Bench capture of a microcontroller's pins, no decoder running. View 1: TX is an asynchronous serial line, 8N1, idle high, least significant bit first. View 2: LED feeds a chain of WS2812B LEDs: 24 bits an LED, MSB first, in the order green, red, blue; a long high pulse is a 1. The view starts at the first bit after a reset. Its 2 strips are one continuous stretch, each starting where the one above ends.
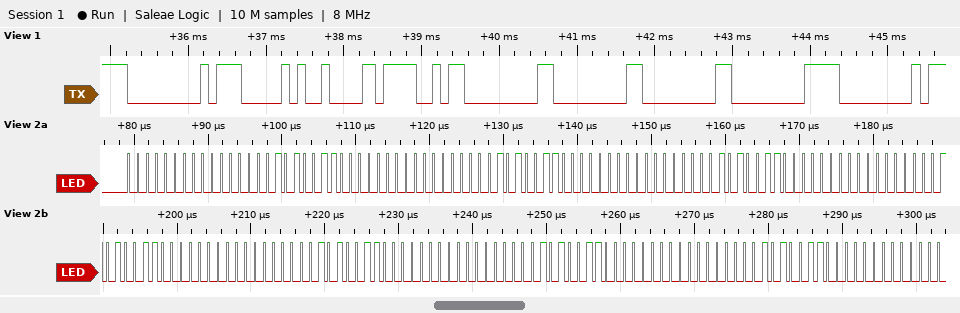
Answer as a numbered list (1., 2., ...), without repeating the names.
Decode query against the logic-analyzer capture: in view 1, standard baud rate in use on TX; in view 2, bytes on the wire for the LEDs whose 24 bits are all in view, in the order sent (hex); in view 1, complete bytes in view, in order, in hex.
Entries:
1. 9600 baud
2. 00 00 A6 00 00 A6 00 00 A6 00 00 A6 00 00 A6 00 00 A6 00 00 A6
3. 00 07 09 4F 00 00 00 00 00
